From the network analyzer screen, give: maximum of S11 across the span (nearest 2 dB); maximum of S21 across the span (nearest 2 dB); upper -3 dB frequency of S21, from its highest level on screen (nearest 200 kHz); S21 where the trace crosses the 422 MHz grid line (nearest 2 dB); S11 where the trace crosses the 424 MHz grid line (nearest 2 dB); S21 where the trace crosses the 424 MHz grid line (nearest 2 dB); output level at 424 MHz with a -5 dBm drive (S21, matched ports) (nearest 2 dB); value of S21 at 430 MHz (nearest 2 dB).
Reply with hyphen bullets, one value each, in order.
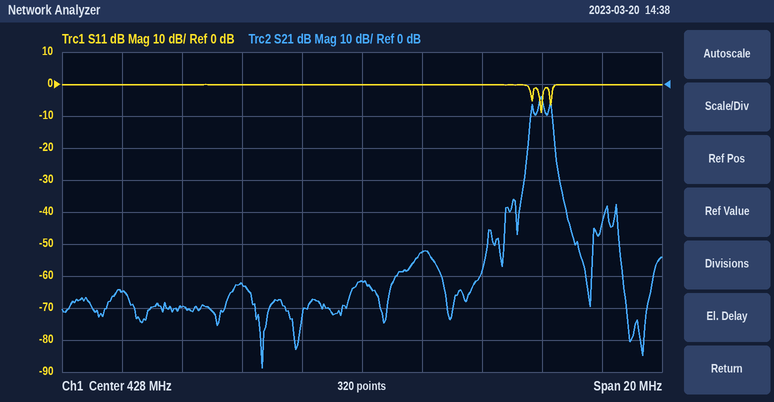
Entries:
- 0 dB
- -4 dB
- 434.0 MHz
- -70 dB
- 0 dB
- -62 dB
- -68 dBm
- -52 dB
